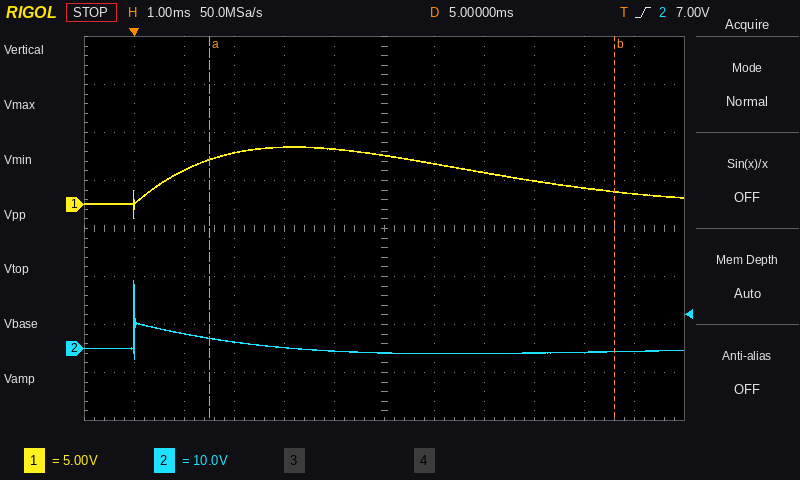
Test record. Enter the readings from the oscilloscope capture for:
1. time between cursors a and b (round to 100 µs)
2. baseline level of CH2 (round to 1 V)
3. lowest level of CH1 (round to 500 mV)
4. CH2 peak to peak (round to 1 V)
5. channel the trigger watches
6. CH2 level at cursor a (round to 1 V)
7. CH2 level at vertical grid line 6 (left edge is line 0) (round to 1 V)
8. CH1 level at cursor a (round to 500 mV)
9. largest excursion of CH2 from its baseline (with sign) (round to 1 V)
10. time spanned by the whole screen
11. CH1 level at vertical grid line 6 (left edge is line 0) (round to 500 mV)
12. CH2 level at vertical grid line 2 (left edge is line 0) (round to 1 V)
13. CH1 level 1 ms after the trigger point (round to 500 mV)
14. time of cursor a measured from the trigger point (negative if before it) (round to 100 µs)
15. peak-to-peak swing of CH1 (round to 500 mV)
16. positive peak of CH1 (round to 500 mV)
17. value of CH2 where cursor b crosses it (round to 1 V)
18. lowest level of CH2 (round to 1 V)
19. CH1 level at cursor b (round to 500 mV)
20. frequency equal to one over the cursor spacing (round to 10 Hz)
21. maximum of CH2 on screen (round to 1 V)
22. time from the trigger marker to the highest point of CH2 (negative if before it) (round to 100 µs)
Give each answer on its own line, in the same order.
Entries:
8.1 ms
-1 V
-1.5 V
16 V
CH2
2 V
-1 V
4.5 V
+15 V
12 ms
5.0 V
3 V
3.5 V
+1.5 ms
7.5 V
6.0 V
-1 V
-2 V
1.5 V
120 Hz
14 V
0.0 ms
